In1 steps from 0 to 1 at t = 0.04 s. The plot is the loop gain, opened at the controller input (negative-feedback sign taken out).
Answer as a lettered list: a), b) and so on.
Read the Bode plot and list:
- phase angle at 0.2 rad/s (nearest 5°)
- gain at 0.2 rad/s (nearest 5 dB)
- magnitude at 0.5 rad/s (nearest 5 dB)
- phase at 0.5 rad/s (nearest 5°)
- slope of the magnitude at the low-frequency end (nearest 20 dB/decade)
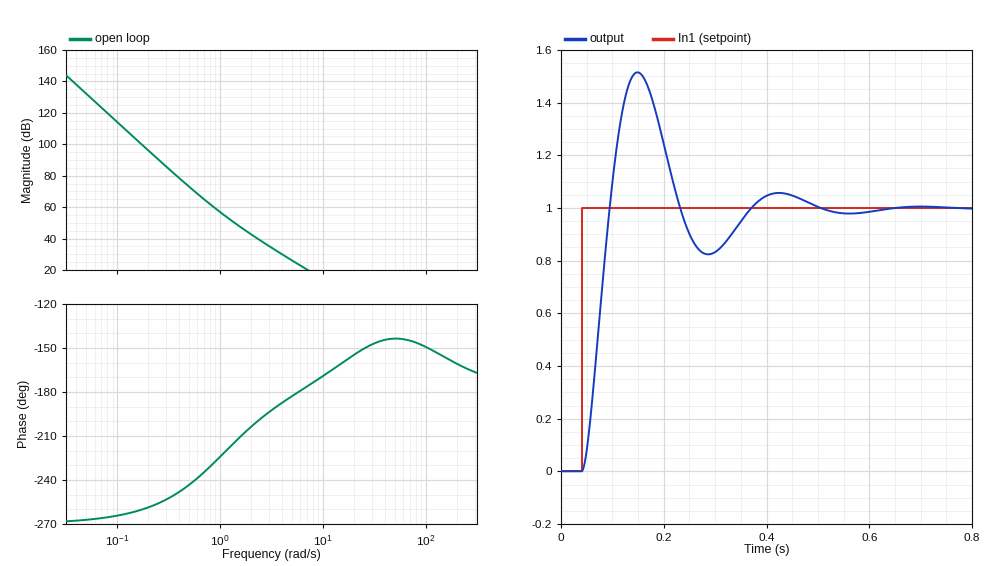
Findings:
a) -260°
b) 95 dB
c) 75 dB
d) -245°
e) -60 dB/decade
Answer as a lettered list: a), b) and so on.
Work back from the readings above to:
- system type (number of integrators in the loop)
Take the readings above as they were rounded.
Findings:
a) 3
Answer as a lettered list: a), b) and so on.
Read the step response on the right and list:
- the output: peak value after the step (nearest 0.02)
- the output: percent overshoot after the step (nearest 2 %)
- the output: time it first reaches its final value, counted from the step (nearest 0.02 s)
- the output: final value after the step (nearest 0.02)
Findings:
a) 1.52
b) 52 %
c) 0.06 s
d) 1.00
